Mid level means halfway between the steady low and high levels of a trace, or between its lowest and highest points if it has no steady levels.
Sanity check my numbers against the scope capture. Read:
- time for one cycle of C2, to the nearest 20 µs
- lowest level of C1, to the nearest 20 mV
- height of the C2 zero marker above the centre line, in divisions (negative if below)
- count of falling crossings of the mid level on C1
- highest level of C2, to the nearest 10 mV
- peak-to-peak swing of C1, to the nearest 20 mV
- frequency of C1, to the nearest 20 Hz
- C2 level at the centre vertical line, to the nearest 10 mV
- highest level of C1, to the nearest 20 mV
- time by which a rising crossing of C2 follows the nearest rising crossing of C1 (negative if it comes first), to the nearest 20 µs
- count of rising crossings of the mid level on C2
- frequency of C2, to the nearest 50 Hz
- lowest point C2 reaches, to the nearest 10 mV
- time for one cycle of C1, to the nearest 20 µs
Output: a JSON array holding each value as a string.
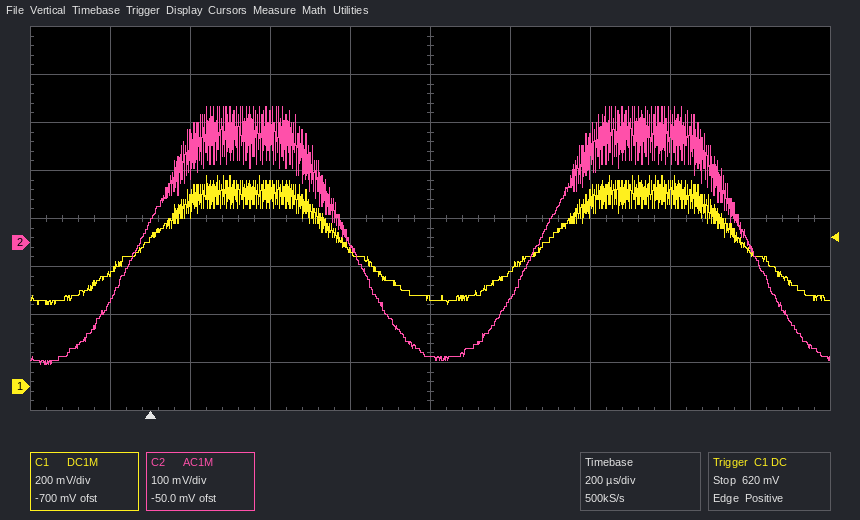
["1.00 ms", "340 mV", "-0.5 div", "2", "280 mV", "540 mV", "1.00 kHz", "-240 mV", "880 mV", "-20 µs", "2", "1.00 kHz", "-250 mV", "1.00 ms"]
